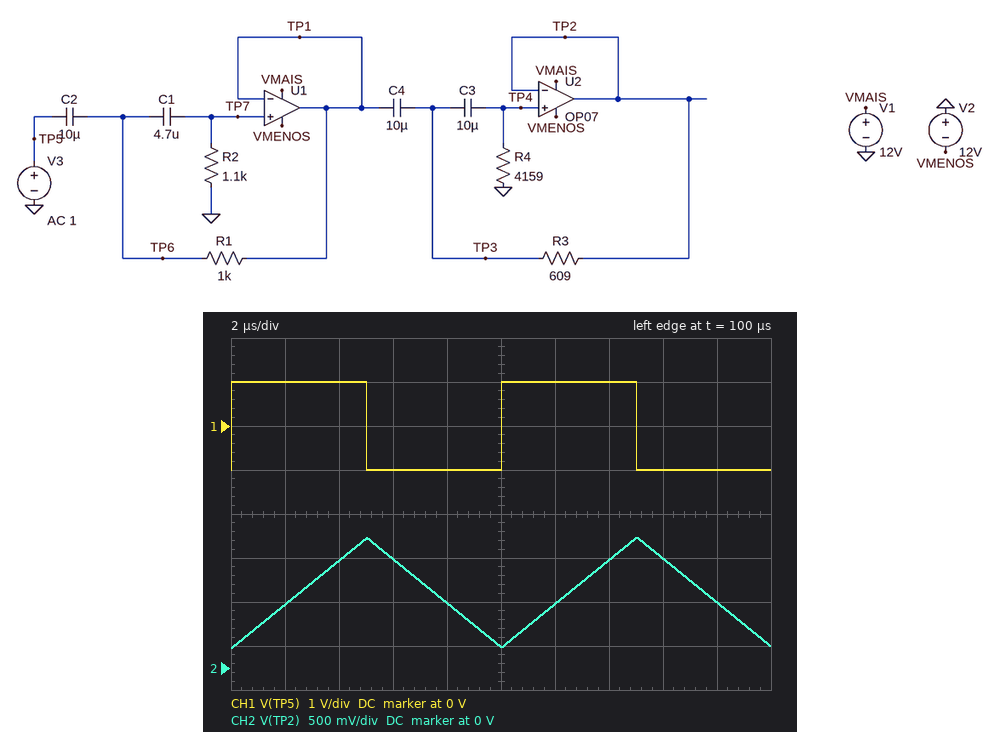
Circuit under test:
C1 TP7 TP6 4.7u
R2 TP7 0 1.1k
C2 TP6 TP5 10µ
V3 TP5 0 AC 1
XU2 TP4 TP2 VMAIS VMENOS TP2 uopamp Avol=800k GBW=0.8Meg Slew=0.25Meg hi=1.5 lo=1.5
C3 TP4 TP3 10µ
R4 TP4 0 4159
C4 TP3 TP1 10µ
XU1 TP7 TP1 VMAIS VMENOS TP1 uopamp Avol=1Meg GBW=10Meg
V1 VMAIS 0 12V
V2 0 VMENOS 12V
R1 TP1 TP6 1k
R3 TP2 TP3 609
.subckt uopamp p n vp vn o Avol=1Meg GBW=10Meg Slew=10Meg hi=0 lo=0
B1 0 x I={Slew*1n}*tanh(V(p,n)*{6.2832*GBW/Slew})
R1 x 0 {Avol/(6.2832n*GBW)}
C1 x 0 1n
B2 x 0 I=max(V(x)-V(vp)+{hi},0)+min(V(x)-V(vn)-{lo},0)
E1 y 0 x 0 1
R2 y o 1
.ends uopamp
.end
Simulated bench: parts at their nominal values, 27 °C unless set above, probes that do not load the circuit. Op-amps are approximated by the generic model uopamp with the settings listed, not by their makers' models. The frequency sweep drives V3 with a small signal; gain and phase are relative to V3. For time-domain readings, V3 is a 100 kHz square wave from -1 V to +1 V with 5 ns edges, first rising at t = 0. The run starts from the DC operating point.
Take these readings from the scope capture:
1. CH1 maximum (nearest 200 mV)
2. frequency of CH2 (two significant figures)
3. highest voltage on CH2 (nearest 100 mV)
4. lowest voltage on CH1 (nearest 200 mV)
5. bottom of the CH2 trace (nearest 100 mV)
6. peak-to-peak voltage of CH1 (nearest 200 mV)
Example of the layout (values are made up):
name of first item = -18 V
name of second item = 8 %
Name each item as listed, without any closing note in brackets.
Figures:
CH1 maximum = 1.0 V
frequency of CH2 = 100 kHz
highest voltage on CH2 = 1.5 V
lowest voltage on CH1 = -1.0 V
bottom of the CH2 trace = 200 mV
peak-to-peak voltage of CH1 = 2.0 V
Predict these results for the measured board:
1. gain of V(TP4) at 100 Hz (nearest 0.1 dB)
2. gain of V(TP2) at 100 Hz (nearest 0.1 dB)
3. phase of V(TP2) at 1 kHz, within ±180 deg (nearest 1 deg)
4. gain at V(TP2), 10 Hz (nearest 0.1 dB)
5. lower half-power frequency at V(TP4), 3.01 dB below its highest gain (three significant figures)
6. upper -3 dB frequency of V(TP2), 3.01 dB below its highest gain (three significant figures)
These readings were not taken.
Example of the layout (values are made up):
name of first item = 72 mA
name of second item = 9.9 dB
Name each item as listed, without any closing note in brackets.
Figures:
gain of V(TP4) at 100 Hz = -0.4 dB
gain of V(TP2) at 100 Hz = -0.4 dB
phase of V(TP2) at 1 kHz, within ±180 deg = 3 deg
gain at V(TP2), 10 Hz = -13.2 dB
lower half-power frequency at V(TP4), 3.01 dB below its highest gain = 31.7 Hz
upper -3 dB frequency of V(TP2), 3.01 dB below its highest gain = 794 kHz
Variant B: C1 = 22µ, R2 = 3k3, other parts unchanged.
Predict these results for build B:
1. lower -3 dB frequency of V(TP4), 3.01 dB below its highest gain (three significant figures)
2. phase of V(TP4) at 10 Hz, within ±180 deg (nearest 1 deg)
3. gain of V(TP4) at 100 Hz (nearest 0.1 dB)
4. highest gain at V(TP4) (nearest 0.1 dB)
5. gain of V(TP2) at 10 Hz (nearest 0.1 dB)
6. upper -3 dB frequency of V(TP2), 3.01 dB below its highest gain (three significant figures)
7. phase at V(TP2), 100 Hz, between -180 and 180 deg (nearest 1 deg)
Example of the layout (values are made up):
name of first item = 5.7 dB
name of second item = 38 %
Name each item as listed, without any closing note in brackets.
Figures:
lower -3 dB frequency of V(TP4), 3.01 dB below its highest gain = 8.49 Hz
phase of V(TP4) at 10 Hz, within ±180 deg = 137 deg
gain of V(TP4) at 100 Hz = 0.1 dB
highest gain at V(TP4) = 3.4 dB
gain of V(TP2) at 10 Hz = 2.7 dB
upper -3 dB frequency of V(TP2), 3.01 dB below its highest gain = 42.7 Hz
phase at V(TP2), 100 Hz, between -180 and 180 deg = 8 deg
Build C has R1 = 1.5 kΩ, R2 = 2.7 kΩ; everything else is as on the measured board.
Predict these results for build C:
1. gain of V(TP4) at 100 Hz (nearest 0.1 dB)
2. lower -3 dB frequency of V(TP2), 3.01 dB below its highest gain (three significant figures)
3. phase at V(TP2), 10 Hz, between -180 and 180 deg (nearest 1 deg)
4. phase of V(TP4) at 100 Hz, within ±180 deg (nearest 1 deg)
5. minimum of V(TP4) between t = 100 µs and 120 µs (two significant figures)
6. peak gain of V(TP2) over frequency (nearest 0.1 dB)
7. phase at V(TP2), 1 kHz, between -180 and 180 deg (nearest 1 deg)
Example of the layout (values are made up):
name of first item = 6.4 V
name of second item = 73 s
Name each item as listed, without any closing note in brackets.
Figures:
gain of V(TP4) at 100 Hz = 0 dB
lower -3 dB frequency of V(TP2), 3.01 dB below its highest gain = 10.3 Hz
phase at V(TP2), 10 Hz, between -180 and 180 deg = -170 deg
phase of V(TP4) at 100 Hz, within ±180 deg = 15 deg
minimum of V(TP4) between t = 100 µs and 120 µs = -24 mV
peak gain of V(TP2) over frequency = 0.4 dB
phase at V(TP2), 1 kHz, between -180 and 180 deg = 1 deg
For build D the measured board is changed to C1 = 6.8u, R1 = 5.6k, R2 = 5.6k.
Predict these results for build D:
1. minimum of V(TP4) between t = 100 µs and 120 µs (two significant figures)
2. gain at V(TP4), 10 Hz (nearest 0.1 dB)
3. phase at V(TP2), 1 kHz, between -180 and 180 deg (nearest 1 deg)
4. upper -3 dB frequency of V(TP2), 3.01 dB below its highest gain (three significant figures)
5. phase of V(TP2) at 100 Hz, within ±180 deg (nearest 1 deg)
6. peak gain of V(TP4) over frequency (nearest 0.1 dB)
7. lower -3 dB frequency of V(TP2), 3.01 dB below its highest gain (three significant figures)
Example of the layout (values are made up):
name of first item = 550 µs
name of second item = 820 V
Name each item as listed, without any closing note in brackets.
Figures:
minimum of V(TP4) between t = 100 µs and 120 µs = -16 mV
gain at V(TP4), 10 Hz = 1.3 dB
phase at V(TP2), 1 kHz, between -180 and 180 deg = 1 deg
upper -3 dB frequency of V(TP2), 3.01 dB below its highest gain = 337 kHz
phase of V(TP2) at 100 Hz, within ±180 deg = 8 deg
peak gain of V(TP4) over frequency = 2.3 dB
lower -3 dB frequency of V(TP2), 3.01 dB below its highest gain = 8.73 Hz
